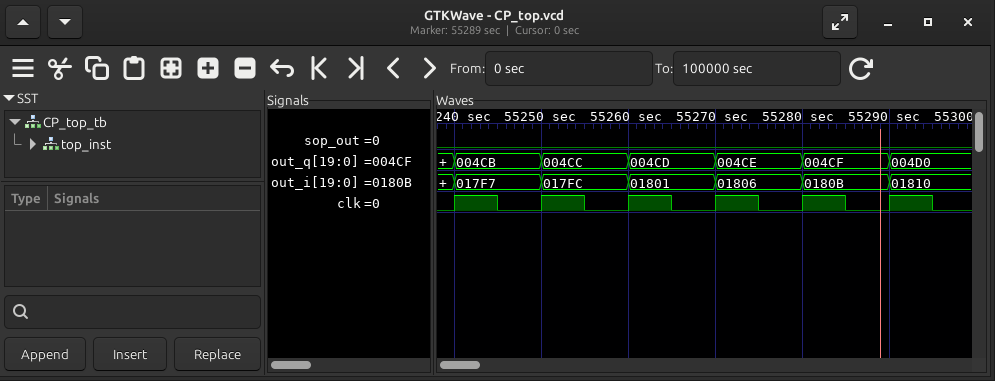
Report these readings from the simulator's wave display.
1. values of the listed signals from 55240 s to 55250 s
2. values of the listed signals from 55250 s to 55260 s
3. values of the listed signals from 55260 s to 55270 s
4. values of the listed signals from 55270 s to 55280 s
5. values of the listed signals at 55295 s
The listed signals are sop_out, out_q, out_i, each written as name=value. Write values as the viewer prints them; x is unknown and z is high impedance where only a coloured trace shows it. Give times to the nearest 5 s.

sop_out=0, out_q=004CB, out_i=017F7
sop_out=0, out_q=004CC, out_i=017FC
sop_out=0, out_q=004CD, out_i=01801
sop_out=0, out_q=004CE, out_i=01806
sop_out=0, out_q=004D0, out_i=01810
